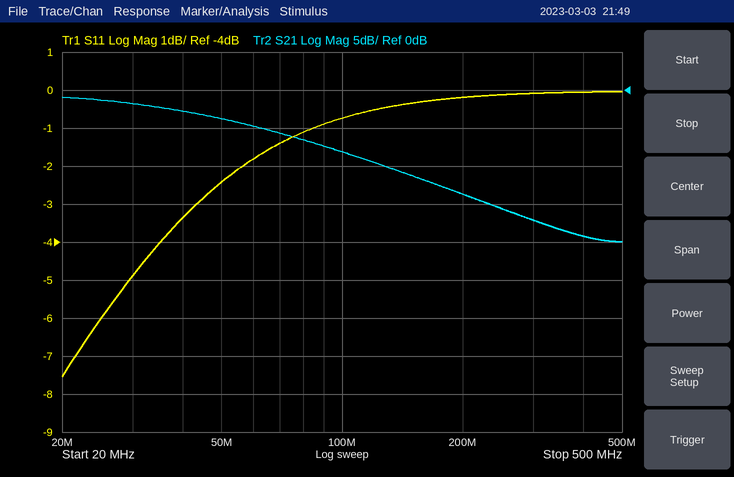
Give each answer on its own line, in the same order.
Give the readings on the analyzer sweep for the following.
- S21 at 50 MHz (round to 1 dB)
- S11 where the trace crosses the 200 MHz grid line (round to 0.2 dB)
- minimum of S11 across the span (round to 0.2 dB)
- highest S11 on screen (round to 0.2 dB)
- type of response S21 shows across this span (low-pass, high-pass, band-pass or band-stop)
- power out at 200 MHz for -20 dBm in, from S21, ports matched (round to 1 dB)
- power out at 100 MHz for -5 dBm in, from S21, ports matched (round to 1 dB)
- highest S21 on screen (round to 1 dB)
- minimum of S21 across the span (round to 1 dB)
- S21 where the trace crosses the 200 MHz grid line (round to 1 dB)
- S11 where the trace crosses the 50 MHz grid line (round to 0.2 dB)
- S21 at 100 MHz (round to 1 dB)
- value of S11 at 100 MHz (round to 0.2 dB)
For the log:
-4 dB
-0.2 dB
-7.6 dB
0.0 dB
low-pass
-34 dBm
-13 dBm
-1 dB
-20 dB
-14 dB
-2.4 dB
-8 dB
-0.8 dB
